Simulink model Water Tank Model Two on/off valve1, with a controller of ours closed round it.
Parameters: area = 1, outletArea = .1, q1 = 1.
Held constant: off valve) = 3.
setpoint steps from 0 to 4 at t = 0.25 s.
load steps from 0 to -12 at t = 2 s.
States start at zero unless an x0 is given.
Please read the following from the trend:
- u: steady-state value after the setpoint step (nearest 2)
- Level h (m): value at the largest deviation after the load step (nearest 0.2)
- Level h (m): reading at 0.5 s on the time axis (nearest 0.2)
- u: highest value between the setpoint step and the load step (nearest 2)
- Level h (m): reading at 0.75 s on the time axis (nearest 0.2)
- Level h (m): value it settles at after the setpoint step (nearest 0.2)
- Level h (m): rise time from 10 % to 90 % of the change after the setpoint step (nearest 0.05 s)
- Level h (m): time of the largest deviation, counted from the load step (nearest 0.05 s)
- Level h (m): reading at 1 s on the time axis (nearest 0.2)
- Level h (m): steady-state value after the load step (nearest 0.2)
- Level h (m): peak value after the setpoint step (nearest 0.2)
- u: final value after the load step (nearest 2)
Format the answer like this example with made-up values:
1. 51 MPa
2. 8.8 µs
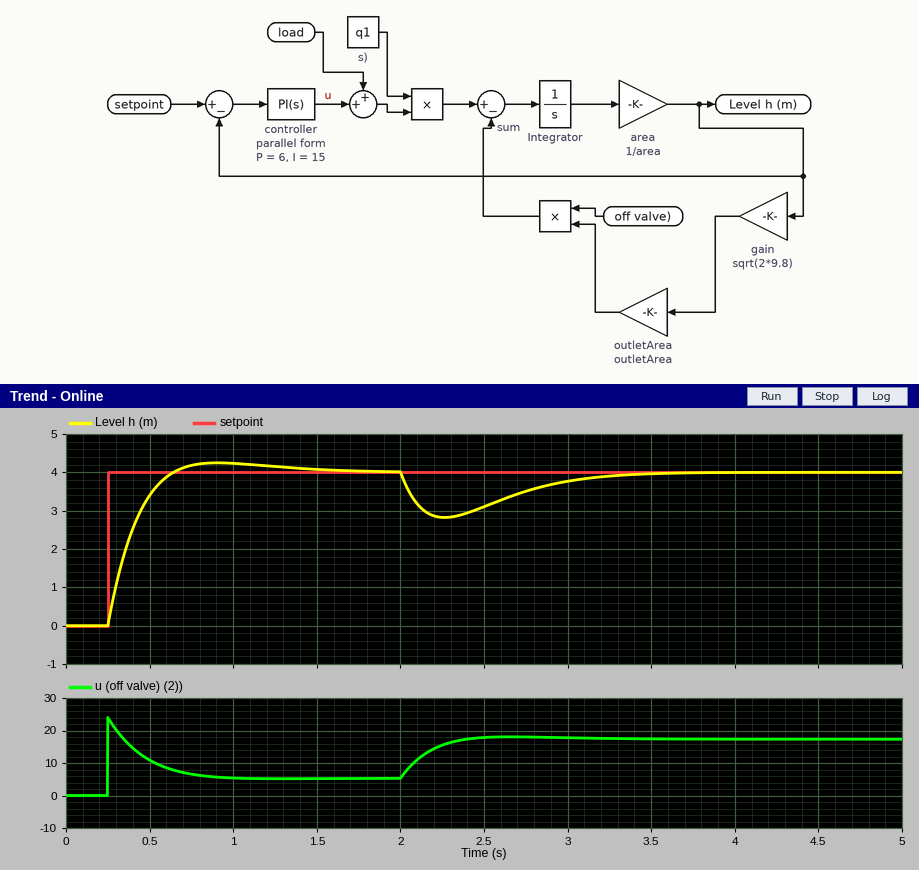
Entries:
1. 6
2. 2.8
3. 3.4
4. 24
5. 4.2
6. 4.0
7. 0.25 s
8. 0.25 s
9. 4.2
10. 4.0
11. 4.2
12. 18
